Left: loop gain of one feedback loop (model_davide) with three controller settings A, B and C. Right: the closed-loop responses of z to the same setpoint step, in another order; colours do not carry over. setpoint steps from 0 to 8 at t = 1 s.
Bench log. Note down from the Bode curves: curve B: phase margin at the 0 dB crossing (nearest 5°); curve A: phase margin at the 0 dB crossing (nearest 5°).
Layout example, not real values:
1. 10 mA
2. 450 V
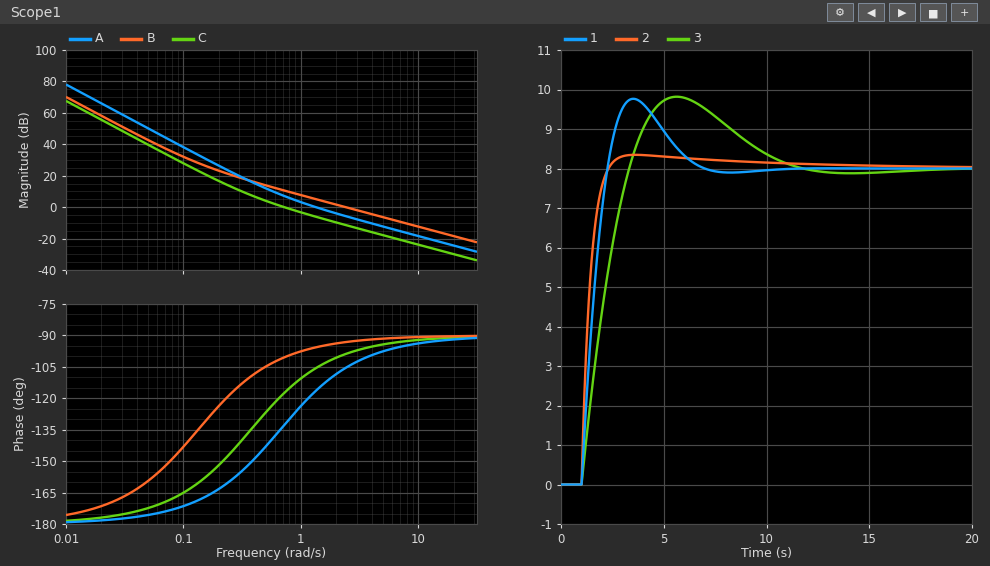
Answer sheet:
1. 85°
2. 65°
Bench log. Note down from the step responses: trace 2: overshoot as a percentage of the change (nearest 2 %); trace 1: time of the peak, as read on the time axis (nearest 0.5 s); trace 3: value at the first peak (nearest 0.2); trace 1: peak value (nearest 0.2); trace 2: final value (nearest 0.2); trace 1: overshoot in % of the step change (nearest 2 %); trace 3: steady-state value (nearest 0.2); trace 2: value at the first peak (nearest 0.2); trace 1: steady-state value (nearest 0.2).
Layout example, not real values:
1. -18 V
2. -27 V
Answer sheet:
1. 4 %
2. 3.5 s
3. 9.8
4. 9.8
5. 8.0
6. 22 %
7. 8.0
8. 8.4
9. 8.0
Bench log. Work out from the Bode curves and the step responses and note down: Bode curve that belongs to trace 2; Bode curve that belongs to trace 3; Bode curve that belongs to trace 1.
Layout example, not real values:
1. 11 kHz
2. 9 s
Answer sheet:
1. B
2. C
3. A
